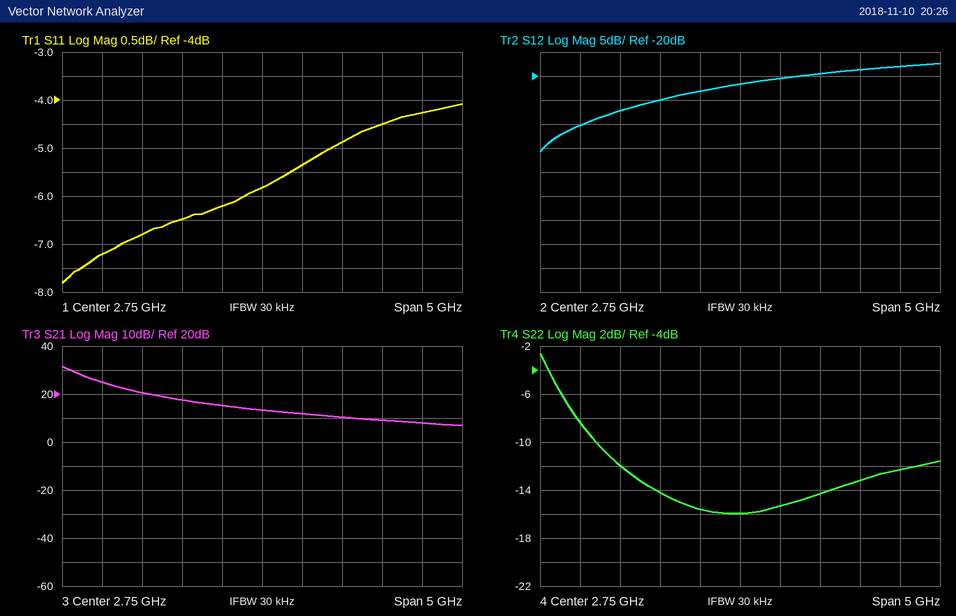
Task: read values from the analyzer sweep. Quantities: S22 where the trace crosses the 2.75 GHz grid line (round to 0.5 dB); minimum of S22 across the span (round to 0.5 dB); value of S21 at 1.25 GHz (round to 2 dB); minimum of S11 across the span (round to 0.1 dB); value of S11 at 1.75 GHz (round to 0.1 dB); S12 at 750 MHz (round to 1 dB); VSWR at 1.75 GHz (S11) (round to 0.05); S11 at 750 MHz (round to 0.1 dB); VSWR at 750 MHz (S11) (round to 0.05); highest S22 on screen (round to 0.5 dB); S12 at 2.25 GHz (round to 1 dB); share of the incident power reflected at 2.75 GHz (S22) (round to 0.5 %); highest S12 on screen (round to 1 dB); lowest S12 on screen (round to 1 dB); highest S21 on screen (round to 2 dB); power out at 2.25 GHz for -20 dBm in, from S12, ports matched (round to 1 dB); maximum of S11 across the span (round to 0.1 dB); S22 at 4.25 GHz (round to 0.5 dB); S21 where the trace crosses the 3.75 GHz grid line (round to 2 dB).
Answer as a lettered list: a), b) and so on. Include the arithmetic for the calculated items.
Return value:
a) -16.0 dB
b) -16.0 dB
c) 20 dB
d) -7.8 dB
e) -6.5 dB
f) -30 dB
g) |Γ| = 10^(-6.5/20) = 0.4732; VSWR = (1 + 0.4732)/(1 − 0.4732) ≈ 2.80
h) -7.2 dB
i) |Γ| = 10^(-7.2/20) = 0.4365; VSWR = (1 + 0.4365)/(1 − 0.4365) ≈ 2.55
j) -2.5 dB
k) -23 dB
l) 10^(-16/10) ≈ 2.5 %
m) -17 dB
n) -36 dB
o) 32 dB
p) -20 dBm + (-23 dB) = -43 dBm
q) -4.1 dB
r) -13.0 dB
s) 10 dB
